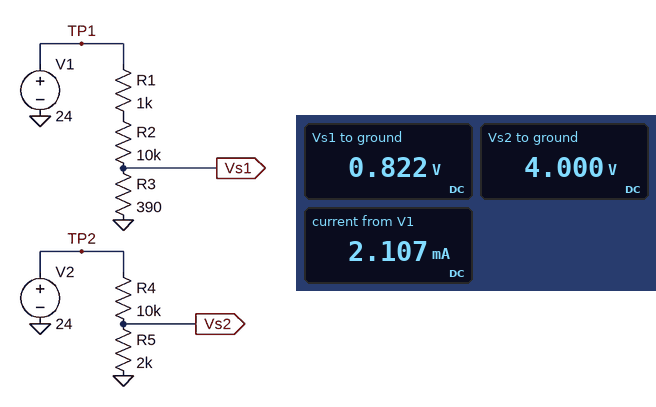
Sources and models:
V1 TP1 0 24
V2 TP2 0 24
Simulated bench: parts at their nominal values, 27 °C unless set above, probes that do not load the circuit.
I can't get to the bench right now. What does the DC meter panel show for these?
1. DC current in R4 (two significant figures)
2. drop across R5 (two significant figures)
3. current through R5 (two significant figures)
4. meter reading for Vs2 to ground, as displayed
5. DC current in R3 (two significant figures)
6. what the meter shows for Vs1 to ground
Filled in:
2.0 mA
4.0 V
2.0 mA
4.000 V
2.1 mA
0.822 V
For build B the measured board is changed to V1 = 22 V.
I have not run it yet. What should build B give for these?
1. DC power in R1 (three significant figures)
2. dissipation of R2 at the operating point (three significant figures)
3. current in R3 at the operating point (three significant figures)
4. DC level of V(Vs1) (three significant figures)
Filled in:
3.73 mW
37.3 mW
1.93 mA
753 mV
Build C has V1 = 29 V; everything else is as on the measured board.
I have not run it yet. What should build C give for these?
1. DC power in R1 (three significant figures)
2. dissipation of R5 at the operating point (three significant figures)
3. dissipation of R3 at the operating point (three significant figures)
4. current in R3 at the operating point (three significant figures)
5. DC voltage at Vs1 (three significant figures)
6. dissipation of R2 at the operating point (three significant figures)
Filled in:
6.48 mW
8.00 mW
2.53 mW
2.55 mA
993 mV
64.8 mW
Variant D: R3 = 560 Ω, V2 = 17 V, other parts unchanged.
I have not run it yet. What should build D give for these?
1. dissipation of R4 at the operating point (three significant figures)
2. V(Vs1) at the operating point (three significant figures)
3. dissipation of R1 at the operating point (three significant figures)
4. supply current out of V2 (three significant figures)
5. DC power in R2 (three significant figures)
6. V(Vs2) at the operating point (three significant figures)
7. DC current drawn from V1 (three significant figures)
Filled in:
20.1 mW
1.16 V
4.31 mW
1.42 mA
43.1 mW
2.83 V
2.08 mA
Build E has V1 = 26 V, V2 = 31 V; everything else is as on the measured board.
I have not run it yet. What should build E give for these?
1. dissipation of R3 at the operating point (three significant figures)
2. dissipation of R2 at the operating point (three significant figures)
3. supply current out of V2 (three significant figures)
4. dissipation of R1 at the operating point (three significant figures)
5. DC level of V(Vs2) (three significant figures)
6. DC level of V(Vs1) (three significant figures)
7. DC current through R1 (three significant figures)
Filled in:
2.03 mW
52.1 mW
2.58 mA
5.21 mW
5.17 V
890 mV
2.28 mA
